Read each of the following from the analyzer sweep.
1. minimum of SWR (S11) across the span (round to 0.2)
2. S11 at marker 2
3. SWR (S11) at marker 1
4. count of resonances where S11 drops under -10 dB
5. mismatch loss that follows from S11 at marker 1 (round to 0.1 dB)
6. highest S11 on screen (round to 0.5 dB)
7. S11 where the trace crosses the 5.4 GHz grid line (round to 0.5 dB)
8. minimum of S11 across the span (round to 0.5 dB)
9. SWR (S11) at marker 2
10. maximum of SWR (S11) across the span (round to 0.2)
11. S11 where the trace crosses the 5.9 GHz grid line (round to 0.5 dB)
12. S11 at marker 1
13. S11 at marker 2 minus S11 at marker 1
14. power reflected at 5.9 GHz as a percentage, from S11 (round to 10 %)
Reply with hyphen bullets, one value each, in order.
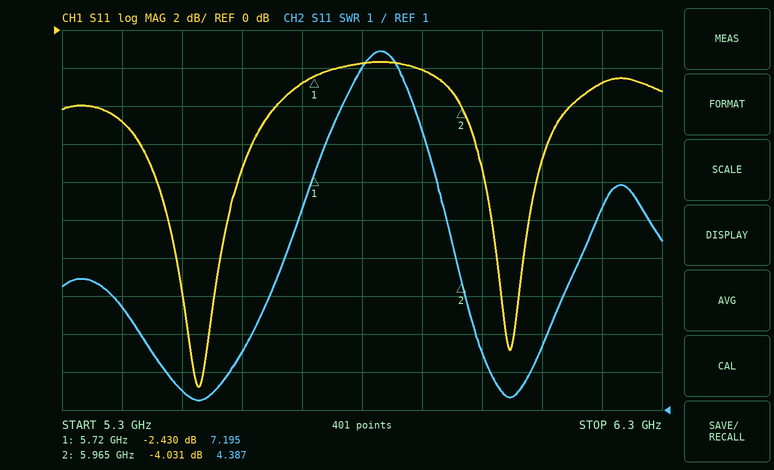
- 1.2
- -4.031 dB
- 7.195
- 2
- 3.7 dB
- -1.5 dB
- -5.0 dB
- -19.0 dB
- 4.387
- 10.4
- -2.0 dB
- -2.430 dB
- -1.601 dB
- 60 %
